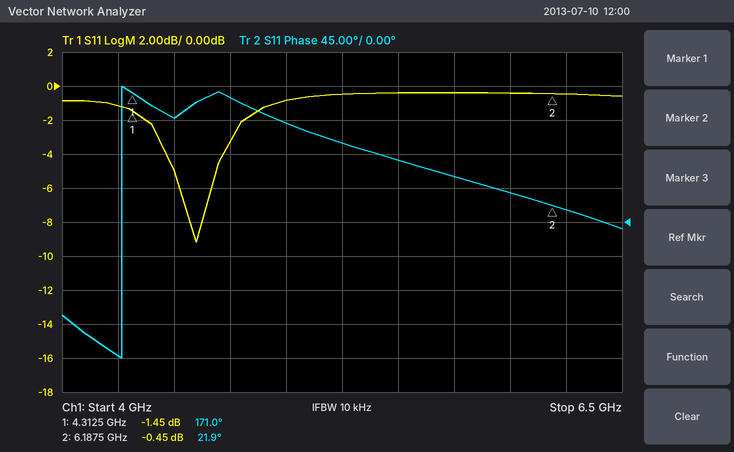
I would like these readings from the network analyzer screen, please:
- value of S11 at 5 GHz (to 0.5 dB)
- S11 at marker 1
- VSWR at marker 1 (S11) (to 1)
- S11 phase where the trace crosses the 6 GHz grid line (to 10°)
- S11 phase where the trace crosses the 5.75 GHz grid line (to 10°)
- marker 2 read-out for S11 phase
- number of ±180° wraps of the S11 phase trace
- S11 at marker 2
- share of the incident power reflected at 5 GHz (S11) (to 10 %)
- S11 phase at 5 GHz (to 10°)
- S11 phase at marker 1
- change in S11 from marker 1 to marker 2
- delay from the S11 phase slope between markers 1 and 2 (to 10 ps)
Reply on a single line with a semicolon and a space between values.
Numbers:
-1.0 dB; -1.45 dB; 12; 40°; 60°; 21.9°; 1; -0.45 dB; 80 %; 130°; 171.0°; 1.00 dB; 220 ps
